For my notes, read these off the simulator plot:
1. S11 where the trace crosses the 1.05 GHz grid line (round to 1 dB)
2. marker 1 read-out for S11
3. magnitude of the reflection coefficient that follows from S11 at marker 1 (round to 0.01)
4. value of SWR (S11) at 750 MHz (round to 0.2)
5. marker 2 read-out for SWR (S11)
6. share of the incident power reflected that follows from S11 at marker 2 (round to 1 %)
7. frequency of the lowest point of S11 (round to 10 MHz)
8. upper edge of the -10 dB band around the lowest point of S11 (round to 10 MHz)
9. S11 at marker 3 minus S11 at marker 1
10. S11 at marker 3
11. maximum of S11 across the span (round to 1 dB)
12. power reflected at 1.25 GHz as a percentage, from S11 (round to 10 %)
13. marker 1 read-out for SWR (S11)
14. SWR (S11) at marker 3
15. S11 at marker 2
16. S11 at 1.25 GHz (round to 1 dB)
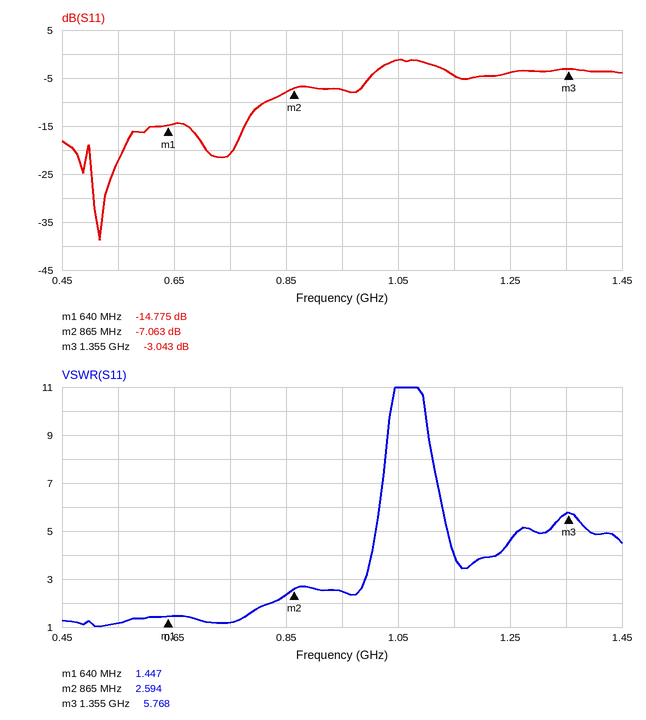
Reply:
-1 dB
-14.775 dB
0.18
1.2
2.594
20 %
520 MHz
810 MHz
11.732 dB
-3.043 dB
-1 dB
40 %
1.447
5.768
-7.063 dB
-4 dB
